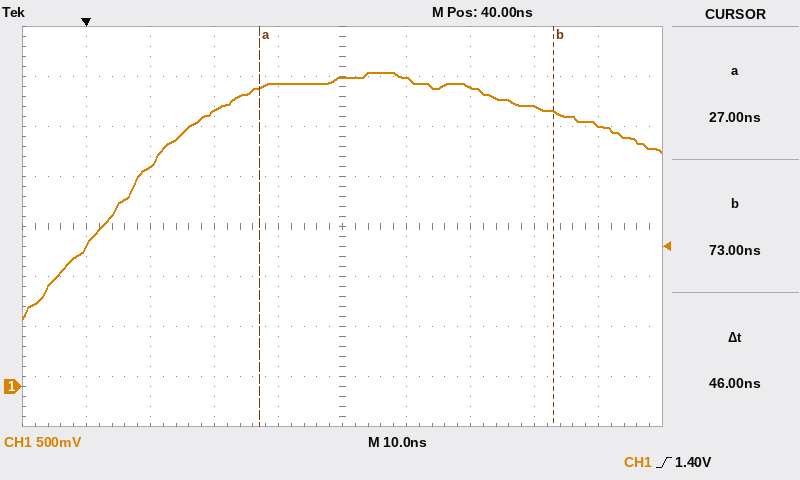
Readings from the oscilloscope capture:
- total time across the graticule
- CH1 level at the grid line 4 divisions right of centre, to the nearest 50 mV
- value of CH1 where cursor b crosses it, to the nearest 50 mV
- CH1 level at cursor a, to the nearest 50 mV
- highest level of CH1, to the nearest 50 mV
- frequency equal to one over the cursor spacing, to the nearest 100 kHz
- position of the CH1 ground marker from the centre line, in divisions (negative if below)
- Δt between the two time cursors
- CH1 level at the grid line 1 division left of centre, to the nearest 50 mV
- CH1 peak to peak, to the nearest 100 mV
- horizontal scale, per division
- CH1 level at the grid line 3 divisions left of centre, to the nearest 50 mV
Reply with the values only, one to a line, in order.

100 ns
2.60 V
2.75 V
3.00 V
3.15 V
21.7 MHz
-3.2 div
46 ns
3.05 V
2.50 V
10 ns
2.20 V
